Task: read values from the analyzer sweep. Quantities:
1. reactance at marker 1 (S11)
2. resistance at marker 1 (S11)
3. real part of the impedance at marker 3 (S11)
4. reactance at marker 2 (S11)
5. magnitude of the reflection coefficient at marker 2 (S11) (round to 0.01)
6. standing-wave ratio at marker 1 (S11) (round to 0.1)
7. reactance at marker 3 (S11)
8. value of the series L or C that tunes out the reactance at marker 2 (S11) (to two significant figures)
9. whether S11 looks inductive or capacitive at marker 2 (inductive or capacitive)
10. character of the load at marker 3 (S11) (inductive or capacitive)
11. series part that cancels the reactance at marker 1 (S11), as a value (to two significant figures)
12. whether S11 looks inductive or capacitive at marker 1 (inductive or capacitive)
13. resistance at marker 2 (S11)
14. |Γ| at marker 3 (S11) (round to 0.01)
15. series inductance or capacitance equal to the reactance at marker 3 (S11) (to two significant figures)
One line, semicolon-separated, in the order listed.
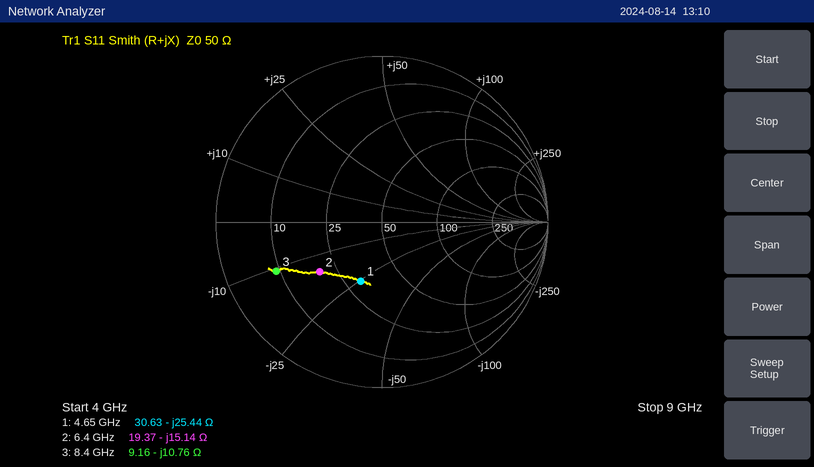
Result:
-25.44 Ω; 30.63 Ω; 9.16 Ω; -15.14 Ω; 0.48; 2.2; -10.76 Ω; 380 pH; capacitive; capacitive; 870 pH; capacitive; 19.37 Ω; 0.70; 1.8 pF
